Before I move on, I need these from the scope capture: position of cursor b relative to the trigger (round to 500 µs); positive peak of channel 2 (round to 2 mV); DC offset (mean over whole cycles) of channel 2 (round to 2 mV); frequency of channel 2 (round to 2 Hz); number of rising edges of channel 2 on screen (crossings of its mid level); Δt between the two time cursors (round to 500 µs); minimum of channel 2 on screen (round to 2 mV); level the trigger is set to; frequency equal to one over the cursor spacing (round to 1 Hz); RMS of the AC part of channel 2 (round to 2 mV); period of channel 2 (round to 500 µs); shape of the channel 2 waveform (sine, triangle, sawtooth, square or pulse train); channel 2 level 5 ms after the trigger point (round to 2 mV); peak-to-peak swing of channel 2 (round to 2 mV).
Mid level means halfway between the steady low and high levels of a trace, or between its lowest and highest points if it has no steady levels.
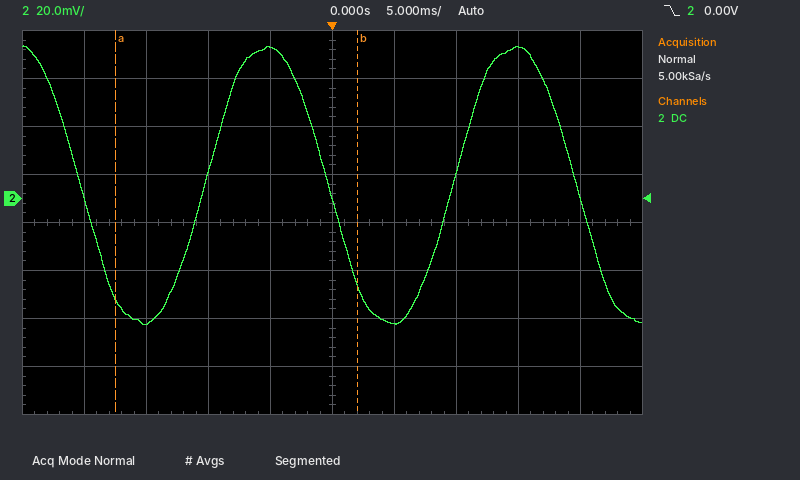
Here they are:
+2.0 ms
64 mV
6 mV
50 Hz
2
19.5 ms
-52 mV
0.00 V
51 Hz
42 mV
20.0 ms
sine
-52 mV
116 mV
